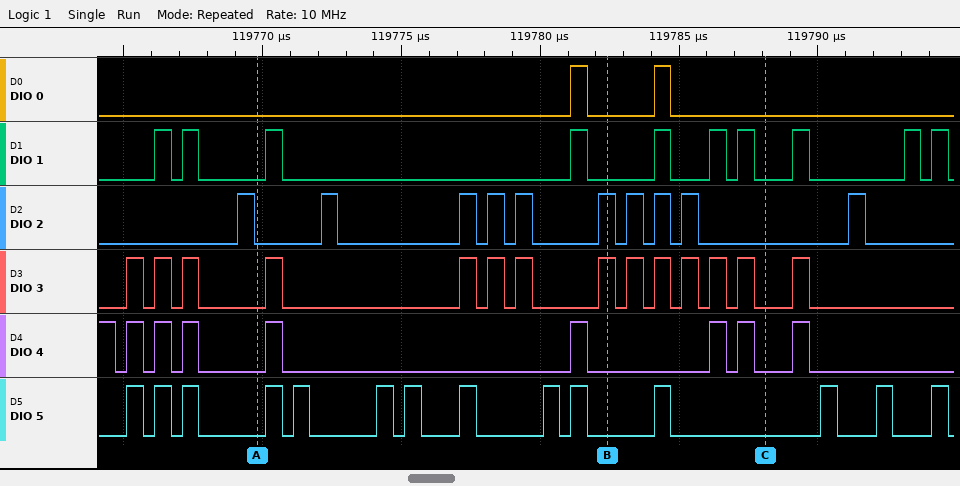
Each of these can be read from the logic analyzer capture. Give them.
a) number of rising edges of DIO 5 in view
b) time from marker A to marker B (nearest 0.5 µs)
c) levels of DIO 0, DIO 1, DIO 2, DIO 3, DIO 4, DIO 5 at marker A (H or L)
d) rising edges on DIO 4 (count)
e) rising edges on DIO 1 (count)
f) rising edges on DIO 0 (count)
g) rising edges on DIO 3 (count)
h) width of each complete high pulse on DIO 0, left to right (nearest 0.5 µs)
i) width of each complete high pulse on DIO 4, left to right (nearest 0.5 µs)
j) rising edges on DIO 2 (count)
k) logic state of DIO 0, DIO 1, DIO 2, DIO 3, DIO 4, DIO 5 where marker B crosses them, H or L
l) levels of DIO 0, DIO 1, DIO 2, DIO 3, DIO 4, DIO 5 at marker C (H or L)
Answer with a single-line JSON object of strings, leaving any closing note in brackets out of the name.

{"number of rising edges of DIO 5 in view": "14", "time from marker A to marker B": "12.5 µs", "levels of DIO 0, DIO 1, DIO 2, DIO 3, DIO 4, DIO 5 at marker A": "DIO 0=L, DIO 1=L, DIO 2=L, DIO 3=L, DIO 4=L, DIO 5=L", "rising edges on DIO 4": "8", "rising edges on DIO 1": "10", "rising edges on DIO 0": "2", "rising edges on DIO 3": "14", "width of each complete high pulse on DIO 0, left to right": "0.5 µs, 0.5 µs", "width of each complete high pulse on DIO 4, left to right": "0.5 µs, 0.5 µs, 0.5 µs, 0.5 µs, 0.5 µs, 0.5 µs, 0.5 µs, 0.5 µs", "rising edges on DIO 2": "10", "logic state of DIO 0, DIO 1, DIO 2, DIO 3, DIO 4, DIO 5 where marker B crosses them, H or L": "DIO 0=L, DIO 1=L, DIO 2=H, DIO 3=H, DIO 4=L, DIO 5=L", "levels of DIO 0, DIO 1, DIO 2, DIO 3, DIO 4, DIO 5 at marker C": "DIO 0=L, DIO 1=L, DIO 2=L, DIO 3=L, DIO 4=L, DIO 5=L"}
